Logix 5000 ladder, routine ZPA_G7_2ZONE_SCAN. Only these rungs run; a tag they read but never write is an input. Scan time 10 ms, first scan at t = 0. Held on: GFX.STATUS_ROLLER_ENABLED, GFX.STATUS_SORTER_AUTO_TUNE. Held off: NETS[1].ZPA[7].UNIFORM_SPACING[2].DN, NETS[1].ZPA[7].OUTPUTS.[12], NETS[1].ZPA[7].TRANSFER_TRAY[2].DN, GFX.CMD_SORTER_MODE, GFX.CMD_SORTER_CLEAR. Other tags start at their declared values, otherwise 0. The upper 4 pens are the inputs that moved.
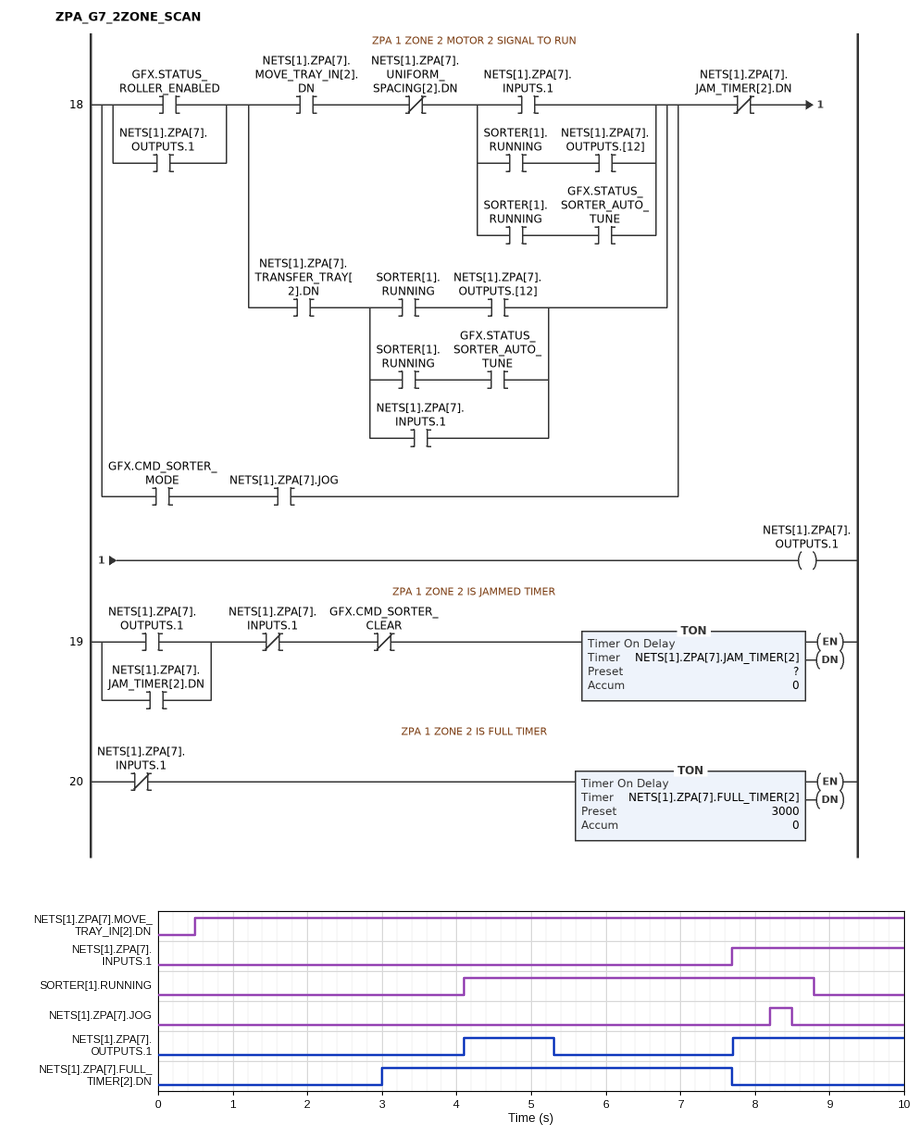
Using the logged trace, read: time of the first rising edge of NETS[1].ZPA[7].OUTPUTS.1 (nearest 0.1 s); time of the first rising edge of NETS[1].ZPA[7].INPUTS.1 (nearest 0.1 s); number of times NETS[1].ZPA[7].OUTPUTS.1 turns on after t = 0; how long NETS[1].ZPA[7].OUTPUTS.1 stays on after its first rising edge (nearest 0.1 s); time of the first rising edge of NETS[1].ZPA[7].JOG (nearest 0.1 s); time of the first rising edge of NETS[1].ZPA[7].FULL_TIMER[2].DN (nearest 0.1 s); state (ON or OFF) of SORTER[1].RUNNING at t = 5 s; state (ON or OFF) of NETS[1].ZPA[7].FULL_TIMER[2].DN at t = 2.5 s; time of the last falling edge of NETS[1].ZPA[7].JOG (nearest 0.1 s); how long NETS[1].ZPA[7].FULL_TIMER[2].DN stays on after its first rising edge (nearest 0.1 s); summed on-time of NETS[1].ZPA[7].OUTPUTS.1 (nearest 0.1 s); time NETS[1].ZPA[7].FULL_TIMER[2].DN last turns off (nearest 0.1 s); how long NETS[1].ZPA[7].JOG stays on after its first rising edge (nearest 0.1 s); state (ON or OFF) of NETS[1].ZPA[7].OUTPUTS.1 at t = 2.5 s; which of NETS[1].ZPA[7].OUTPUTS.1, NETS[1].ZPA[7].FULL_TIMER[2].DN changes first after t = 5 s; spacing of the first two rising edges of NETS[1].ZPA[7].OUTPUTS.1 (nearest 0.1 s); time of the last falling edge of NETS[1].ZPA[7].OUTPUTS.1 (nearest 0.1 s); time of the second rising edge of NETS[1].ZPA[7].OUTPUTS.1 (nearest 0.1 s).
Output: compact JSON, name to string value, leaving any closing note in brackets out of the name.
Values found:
{"time of the first rising edge of NETS[1].ZPA[7].OUTPUTS.1": "4.1 s", "time of the first rising edge of NETS[1].ZPA[7].INPUTS.1": "7.7 s", "number of times NETS[1].ZPA[7].OUTPUTS.1 turns on after t = 0": "2", "how long NETS[1].ZPA[7].OUTPUTS.1 stays on after its first rising edge": "1.2 s", "time of the first rising edge of NETS[1].ZPA[7].JOG": "8.2 s", "time of the first rising edge of NETS[1].ZPA[7].FULL_TIMER[2].DN": "3.0 s", "state (ON or OFF) of SORTER[1].RUNNING at t = 5 s": "ON", "state (ON or OFF) of NETS[1].ZPA[7].FULL_TIMER[2].DN at t = 2.5 s": "OFF", "time of the last falling edge of NETS[1].ZPA[7].JOG": "8.5 s", "how long NETS[1].ZPA[7].FULL_TIMER[2].DN stays on after its first rising edge": "4.7 s", "summed on-time of NETS[1].ZPA[7].OUTPUTS.1": "3.5 s", "time NETS[1].ZPA[7].FULL_TIMER[2].DN last turns off": "7.7 s", "how long NETS[1].ZPA[7].JOG stays on after its first rising edge": "0.3 s", "state (ON or OFF) of NETS[1].ZPA[7].OUTPUTS.1 at t = 2.5 s": "OFF", "which of NETS[1].ZPA[7].OUTPUTS.1, NETS[1].ZPA[7].FULL_TIMER[2].DN changes first after t = 5 s": "NETS[1].ZPA[7].OUTPUTS.1", "spacing of the first two rising edges of NETS[1].ZPA[7].OUTPUTS.1": "3.6 s", "time of the last falling edge of NETS[1].ZPA[7].OUTPUTS.1": "5.3 s", "time of the second rising edge of NETS[1].ZPA[7].OUTPUTS.1": "7.7 s"}
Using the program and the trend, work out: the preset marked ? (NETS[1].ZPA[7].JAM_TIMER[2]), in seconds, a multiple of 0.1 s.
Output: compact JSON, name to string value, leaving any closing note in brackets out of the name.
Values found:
{"the preset marked ? (NETS[1].ZPA[7].JAM_TIMER[2]), in seconds, a multiple of 0.1 s": "1.2 s"}
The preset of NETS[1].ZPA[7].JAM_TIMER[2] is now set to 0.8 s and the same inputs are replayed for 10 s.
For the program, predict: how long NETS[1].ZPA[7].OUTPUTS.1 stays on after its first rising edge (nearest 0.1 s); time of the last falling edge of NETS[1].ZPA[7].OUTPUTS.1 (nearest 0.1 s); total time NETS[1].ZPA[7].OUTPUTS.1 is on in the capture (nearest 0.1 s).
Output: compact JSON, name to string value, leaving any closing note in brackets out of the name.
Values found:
{"how long NETS[1].ZPA[7].OUTPUTS.1 stays on after its first rising edge": "0.8 s", "time of the last falling edge of NETS[1].ZPA[7].OUTPUTS.1": "4.9 s", "total time NETS[1].ZPA[7].OUTPUTS.1 is on in the capture": "3.1 s"}
